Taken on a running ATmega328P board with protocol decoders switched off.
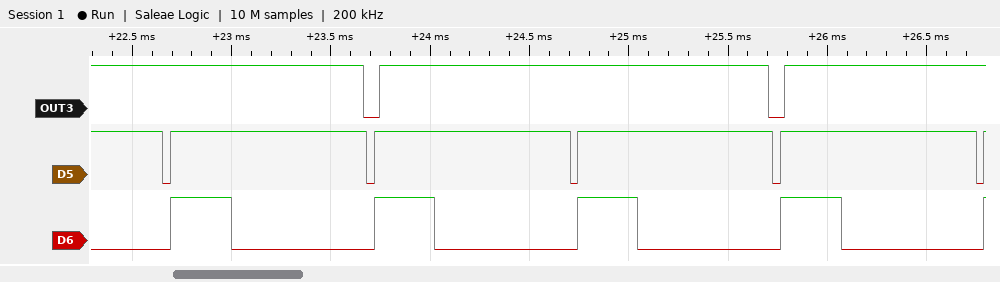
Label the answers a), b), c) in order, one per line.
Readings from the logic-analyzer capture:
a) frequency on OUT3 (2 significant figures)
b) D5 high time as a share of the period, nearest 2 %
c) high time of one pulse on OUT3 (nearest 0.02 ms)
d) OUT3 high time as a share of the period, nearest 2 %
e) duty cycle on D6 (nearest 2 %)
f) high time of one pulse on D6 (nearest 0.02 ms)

a) 490 Hz
b) 96 %
c) 1.96 ms
d) 96 %
e) 30 %
f) 0.30 ms
